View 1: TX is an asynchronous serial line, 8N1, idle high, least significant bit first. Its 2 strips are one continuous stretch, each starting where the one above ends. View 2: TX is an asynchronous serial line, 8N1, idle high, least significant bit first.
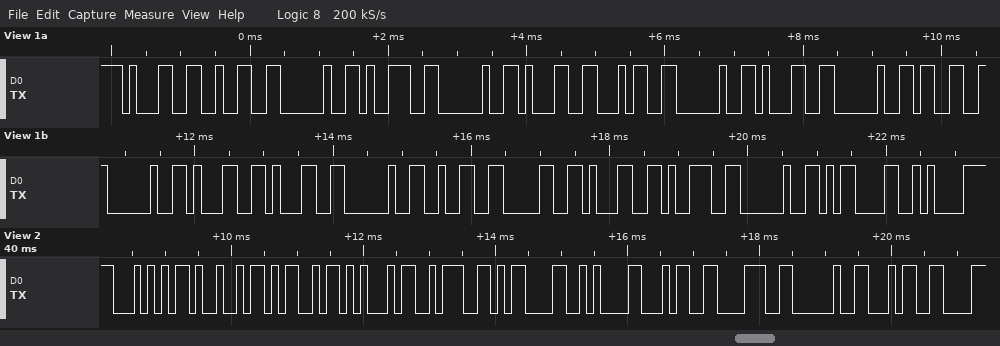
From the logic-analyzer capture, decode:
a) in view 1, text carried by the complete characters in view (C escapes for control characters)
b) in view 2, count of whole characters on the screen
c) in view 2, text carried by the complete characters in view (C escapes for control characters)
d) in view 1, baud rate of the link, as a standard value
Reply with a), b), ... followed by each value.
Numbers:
a) "12 9 14 1 3 11 2019 \r\n"
b) 11
c) "TIME:\r\n48 4"
d) 9600 baud
